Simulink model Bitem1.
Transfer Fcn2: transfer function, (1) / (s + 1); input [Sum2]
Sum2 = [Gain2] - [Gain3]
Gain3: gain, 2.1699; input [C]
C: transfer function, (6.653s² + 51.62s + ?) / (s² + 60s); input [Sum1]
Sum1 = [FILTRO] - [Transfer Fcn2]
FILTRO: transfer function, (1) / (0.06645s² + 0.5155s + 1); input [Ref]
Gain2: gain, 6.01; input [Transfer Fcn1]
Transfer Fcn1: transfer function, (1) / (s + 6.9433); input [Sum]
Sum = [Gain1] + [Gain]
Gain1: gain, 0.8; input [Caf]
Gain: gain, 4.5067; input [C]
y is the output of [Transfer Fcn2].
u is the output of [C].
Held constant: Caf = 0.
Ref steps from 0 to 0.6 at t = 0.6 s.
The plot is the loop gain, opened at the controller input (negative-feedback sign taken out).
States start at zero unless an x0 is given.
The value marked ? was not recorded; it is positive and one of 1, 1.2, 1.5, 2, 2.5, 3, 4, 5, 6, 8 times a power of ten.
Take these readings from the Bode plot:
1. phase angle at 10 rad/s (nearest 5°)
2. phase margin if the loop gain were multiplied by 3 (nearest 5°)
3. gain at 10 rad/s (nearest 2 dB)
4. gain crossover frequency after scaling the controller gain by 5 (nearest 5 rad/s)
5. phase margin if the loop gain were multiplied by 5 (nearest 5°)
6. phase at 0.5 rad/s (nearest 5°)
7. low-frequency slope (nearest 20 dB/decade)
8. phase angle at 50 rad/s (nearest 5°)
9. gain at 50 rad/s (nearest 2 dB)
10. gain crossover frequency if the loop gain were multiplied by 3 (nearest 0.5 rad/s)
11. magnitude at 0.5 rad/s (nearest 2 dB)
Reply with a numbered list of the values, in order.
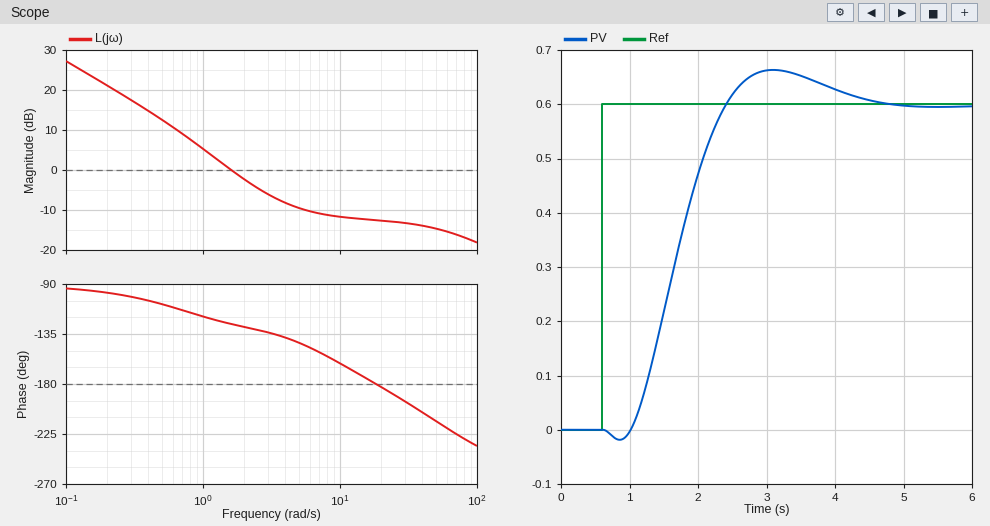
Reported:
1. -160°
2. 35°
3. -12 dB
4. 40 rad/s
5. -25°
6. -110°
7. -20 dB/decade
8. -215°
9. -14 dB
10. 5.0 rad/s
11. 12 dB
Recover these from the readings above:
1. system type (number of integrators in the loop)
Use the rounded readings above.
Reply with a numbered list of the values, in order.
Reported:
1. 1
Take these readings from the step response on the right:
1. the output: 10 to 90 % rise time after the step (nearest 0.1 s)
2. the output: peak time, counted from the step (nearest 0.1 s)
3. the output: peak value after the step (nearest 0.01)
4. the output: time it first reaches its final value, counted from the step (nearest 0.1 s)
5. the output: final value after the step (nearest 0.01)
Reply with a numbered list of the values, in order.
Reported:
1. 1.0 s
2. 2.5 s
3. 0.66
4. 1.8 s
5. 0.60
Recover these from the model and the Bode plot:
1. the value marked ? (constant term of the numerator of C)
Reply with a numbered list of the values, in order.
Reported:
1. 80
